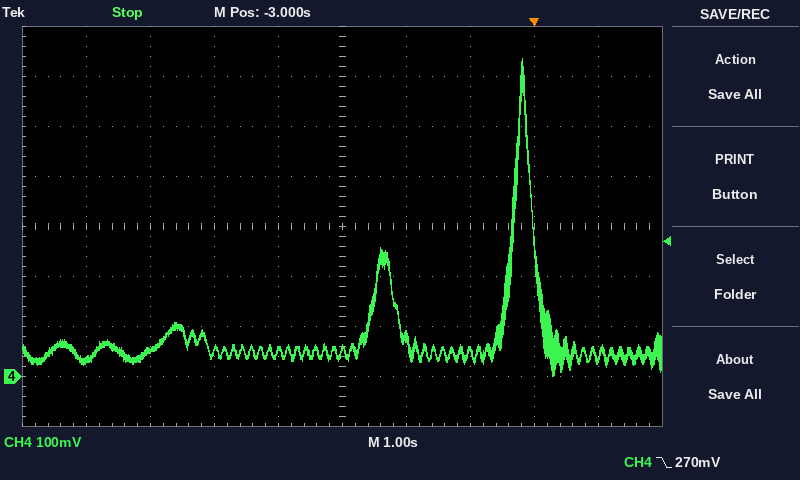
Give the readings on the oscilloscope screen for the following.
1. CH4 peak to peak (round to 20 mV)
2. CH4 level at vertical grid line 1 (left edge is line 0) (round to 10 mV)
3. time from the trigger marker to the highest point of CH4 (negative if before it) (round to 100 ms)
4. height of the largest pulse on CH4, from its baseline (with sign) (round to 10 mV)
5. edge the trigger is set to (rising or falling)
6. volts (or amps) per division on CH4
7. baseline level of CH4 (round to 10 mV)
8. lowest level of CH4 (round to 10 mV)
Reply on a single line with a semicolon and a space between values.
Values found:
640 mV; 30 mV; -200 ms; +580 mV; falling; 100 mV; 50 mV; 0 mV
